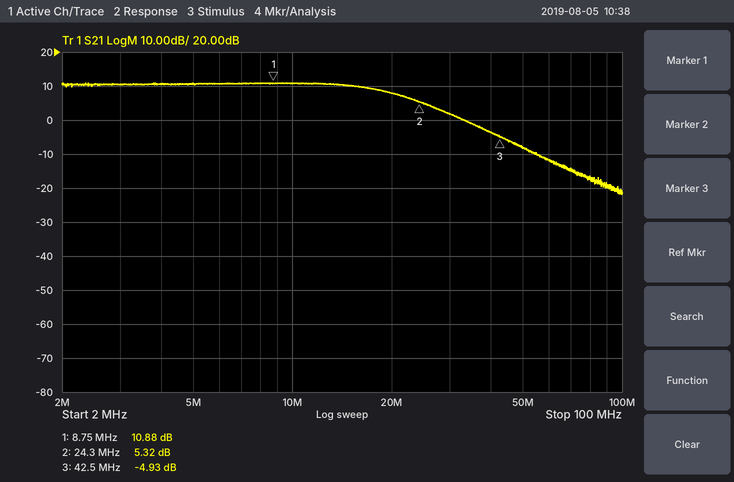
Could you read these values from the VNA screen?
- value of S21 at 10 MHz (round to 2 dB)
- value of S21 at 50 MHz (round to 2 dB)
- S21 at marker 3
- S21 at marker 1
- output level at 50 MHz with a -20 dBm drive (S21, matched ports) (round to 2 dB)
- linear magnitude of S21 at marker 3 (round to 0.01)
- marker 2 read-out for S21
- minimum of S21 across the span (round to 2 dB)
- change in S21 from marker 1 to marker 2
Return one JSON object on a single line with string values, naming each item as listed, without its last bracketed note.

{"value of S21 at 10 MHz": "10 dB", "value of S21 at 50 MHz": "-8 dB", "S21 at marker 3": "-4.93 dB", "S21 at marker 1": "10.88 dB", "output level at 50 MHz with a -20 dBm drive (S21, matched ports)": "-28 dBm", "linear magnitude of S21 at marker 3": "0.57", "marker 2 read-out for S21": "5.32 dB", "minimum of S21 across the span": "-22 dB", "change in S21 from marker 1 to marker 2": "-5.56 dB"}
